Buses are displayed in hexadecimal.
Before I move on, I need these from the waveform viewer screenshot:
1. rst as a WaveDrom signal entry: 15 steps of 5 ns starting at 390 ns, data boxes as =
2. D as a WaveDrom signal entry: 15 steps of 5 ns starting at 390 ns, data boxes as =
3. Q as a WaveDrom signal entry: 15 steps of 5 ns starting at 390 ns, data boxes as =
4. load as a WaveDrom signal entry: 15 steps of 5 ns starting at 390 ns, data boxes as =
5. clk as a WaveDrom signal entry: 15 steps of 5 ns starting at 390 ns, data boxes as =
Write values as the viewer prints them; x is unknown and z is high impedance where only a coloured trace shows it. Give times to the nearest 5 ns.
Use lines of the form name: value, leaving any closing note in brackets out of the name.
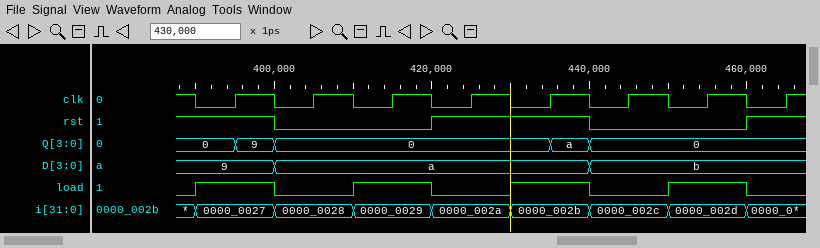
rst as a WaveDrom signal entry: 15 steps of 5 ns starting at 390 ns, data boxes as =: {name: 'rst', wave: '1.0...1...0...1'}
D as a WaveDrom signal entry: 15 steps of 5 ns starting at 390 ns, data boxes as =: {name: 'D', wave: '=.=.......=....', data: '9 a b'}
Q as a WaveDrom signal entry: 15 steps of 5 ns starting at 390 ns, data boxes as =: {name: 'Q', wave: '===......==....', data: '0 9 0 a 0'}
load as a WaveDrom signal entry: 15 steps of 5 ns starting at 390 ns, data boxes as =: {name: 'load', wave: '1.0.1.0.1.0.1.0'}
clk as a WaveDrom signal entry: 15 steps of 5 ns starting at 390 ns, data boxes as =: {name: 'clk', wave: '010101010101010'}
